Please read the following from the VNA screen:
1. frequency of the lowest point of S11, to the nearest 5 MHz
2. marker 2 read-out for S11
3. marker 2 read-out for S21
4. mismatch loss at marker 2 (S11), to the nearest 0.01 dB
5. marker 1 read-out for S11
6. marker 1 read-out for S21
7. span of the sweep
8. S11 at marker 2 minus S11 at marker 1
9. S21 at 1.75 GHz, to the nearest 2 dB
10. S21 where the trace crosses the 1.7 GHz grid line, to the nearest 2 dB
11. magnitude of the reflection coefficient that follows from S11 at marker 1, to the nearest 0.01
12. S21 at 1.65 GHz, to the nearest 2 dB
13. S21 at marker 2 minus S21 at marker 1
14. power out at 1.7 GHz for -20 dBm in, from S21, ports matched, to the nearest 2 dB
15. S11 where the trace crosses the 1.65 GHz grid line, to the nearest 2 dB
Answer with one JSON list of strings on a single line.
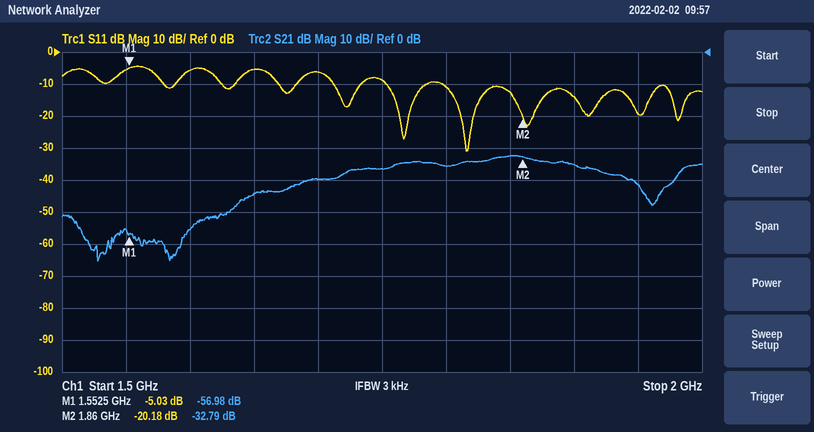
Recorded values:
["1.815 GHz", "-20.18 dB", "-32.79 dB", "0.04 dB", "-5.03 dB", "-56.98 dB", "500 MHz", "-15.15 dB", "-36 dB", "-40 dB", "0.56", "-44 dB", "24.19 dB", "-60 dBm", "-6 dB"]
